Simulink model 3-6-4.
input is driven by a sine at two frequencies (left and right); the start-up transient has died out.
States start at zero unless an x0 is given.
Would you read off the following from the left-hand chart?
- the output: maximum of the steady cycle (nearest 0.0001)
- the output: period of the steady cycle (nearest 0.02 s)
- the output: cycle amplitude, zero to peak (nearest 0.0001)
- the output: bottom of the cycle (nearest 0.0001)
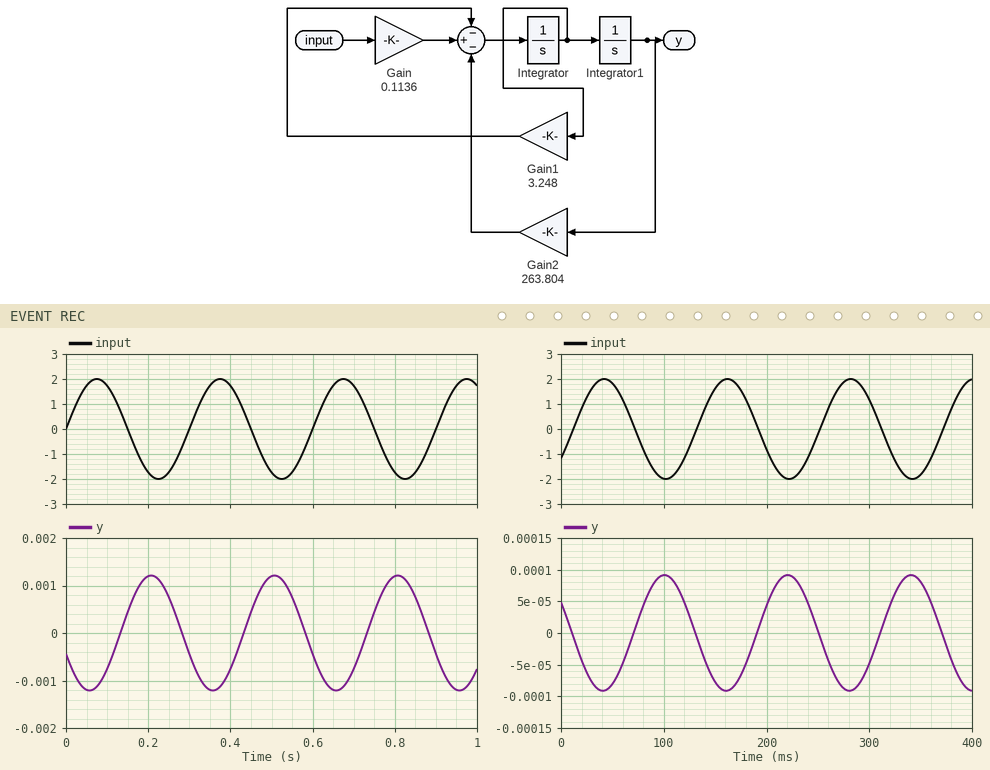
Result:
0.0012
0.30 s
0.0012
-0.0012
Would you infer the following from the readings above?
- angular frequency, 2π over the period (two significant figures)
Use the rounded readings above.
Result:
21 rad/s
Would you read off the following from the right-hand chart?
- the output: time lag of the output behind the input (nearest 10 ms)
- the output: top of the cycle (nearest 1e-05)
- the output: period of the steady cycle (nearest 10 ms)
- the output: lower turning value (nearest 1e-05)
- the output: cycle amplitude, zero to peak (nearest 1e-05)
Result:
60 ms
0.00009
120 ms
-0.00009
0.00009
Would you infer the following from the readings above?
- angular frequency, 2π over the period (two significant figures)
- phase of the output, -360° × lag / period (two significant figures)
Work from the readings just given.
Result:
0.052 rad/ms
-180°
